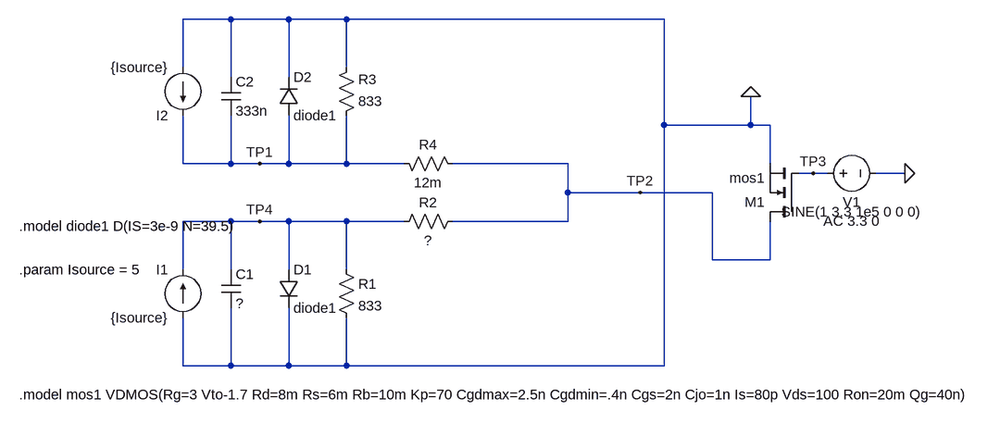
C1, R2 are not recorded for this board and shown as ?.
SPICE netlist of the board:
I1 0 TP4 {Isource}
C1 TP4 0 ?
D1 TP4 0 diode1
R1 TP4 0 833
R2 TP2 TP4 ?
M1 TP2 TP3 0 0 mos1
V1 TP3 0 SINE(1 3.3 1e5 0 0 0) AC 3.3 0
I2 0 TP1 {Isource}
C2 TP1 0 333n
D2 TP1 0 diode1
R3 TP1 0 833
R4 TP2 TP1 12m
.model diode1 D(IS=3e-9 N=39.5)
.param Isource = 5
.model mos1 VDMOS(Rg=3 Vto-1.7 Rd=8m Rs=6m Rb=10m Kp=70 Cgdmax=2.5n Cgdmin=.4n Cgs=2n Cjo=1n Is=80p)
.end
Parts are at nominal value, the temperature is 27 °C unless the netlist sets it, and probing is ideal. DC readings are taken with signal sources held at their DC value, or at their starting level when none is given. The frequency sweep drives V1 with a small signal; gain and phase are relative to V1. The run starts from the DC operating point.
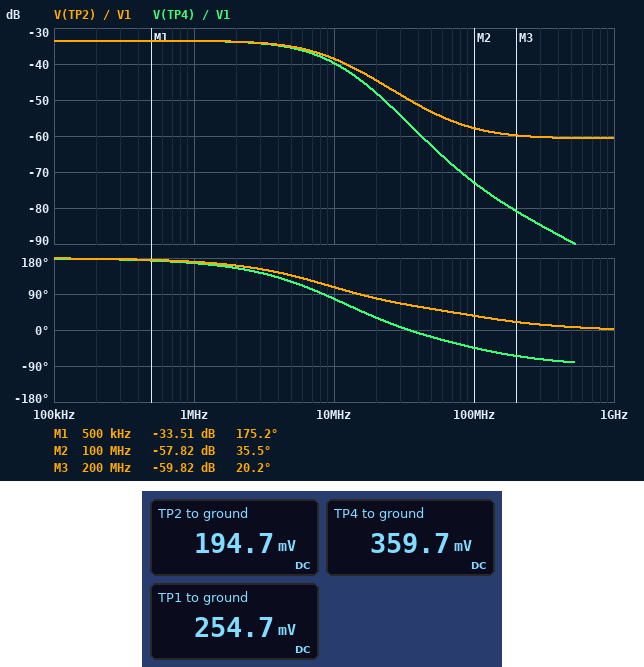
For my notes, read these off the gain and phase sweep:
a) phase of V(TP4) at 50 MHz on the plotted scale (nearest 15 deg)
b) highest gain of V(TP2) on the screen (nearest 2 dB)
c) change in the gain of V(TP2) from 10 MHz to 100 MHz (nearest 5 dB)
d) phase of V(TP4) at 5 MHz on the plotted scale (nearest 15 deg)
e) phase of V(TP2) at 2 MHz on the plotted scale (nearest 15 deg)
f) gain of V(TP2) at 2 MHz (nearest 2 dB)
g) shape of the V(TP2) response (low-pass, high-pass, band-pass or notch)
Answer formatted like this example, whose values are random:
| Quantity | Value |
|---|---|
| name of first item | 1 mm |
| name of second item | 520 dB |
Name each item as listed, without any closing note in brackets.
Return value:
| Quantity | Value |
|---|---|
| phase of V(TP4) at 50 MHz on the plotted scale | -15 deg |
| highest gain of V(TP2) on the screen | -34 dB |
| change in the gain of V(TP2) from 10 MHz to 100 MHz | -20 dB |
| phase of V(TP4) at 5 MHz on the plotted scale | 120 deg |
| phase of V(TP2) at 2 MHz on the plotted scale | 165 deg |
| gain of V(TP2) at 2 MHz | -34 dB |
| shape of the V(TP2) response | low-pass |
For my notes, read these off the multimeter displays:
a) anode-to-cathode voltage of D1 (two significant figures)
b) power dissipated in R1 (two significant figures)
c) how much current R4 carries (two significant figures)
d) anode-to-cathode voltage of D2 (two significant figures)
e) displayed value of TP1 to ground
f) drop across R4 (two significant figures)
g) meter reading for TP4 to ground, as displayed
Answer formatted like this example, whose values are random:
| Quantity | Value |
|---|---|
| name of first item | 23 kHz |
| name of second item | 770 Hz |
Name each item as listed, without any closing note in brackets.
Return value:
| Quantity | Value |
|---|---|
| anode-to-cathode voltage of D1 | 360 mV |
| power dissipated in R1 | 160 µW |
| how much current R4 carries | 5.0 A |
| anode-to-cathode voltage of D2 | 250 mV |
| displayed value of TP1 to ground | 254.7 mV |
| drop across R4 | 60 mV |
| meter reading for TP4 to ground, as displayed | 359.7 mV |
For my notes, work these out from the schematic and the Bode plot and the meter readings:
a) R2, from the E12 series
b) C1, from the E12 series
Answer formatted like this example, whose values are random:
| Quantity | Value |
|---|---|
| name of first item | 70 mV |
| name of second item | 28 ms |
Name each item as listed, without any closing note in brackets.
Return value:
| Quantity | Value |
|---|---|
| R2, from the E12 series | 0.033 Ω |
| C1, from the E12 series | 270 nF |
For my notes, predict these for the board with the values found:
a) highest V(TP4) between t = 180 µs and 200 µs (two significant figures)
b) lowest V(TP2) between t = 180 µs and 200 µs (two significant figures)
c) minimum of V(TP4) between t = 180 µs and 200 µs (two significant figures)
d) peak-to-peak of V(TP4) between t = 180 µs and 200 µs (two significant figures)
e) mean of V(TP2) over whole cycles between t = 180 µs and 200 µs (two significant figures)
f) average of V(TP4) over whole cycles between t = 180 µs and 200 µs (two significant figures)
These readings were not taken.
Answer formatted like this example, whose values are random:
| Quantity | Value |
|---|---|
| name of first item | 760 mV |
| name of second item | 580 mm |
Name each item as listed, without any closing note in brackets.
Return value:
| Quantity | Value |
|---|---|
| highest V(TP4) between t = 180 µs and 200 µs | 22 V |
| lowest V(TP2) between t = 180 µs and 200 µs | 160 mV |
| minimum of V(TP4) between t = 180 µs and 200 µs | 330 mV |
| peak-to-peak of V(TP4) between t = 180 µs and 200 µs | 21 V |
| mean of V(TP2) over whole cycles between t = 180 µs and 200 µs | 5.3 V |
| average of V(TP4) over whole cycles between t = 180 µs and 200 µs | 5.5 V |
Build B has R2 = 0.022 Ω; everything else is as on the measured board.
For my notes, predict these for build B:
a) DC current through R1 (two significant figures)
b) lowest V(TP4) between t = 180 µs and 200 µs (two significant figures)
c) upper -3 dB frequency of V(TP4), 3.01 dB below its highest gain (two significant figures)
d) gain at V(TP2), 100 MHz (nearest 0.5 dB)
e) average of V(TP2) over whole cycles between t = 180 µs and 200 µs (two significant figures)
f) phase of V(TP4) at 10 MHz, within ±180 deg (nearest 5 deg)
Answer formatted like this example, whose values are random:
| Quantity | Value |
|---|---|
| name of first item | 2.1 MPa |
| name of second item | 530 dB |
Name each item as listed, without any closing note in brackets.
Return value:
| Quantity | Value |
|---|---|
| DC current through R1 | 370 µA |
| lowest V(TP4) between t = 180 µs and 200 µs | 270 mV |
| upper -3 dB frequency of V(TP4), 3.01 dB below its highest gain | 6.8 MHz |
| gain at V(TP2), 100 MHz | -58.5 dB |
| average of V(TP2) over whole cycles between t = 180 µs and 200 µs | 5.3 V |
| phase of V(TP4) at 10 MHz, within ±180 deg | 85 deg |
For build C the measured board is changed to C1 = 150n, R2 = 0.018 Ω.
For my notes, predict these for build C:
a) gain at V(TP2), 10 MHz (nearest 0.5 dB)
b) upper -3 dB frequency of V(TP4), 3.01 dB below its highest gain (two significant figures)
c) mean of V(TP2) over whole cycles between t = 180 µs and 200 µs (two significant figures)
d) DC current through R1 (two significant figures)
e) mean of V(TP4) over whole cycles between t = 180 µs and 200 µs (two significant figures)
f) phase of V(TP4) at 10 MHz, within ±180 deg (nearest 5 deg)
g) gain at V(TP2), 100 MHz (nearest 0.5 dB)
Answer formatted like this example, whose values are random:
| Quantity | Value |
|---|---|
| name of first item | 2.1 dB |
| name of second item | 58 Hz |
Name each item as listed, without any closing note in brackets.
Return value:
| Quantity | Value |
|---|---|
| gain at V(TP2), 10 MHz | -37.5 dB |
| upper -3 dB frequency of V(TP4), 3.01 dB below its highest gain | 8.0 MHz |
| mean of V(TP2) over whole cycles between t = 180 µs and 200 µs | 5.5 V |
| DC current through R1 | 340 µA |
| mean of V(TP4) over whole cycles between t = 180 µs and 200 µs | 5.6 V |
| phase of V(TP4) at 10 MHz, within ±180 deg | 100 deg |
| gain at V(TP2), 100 MHz | -58.5 dB |
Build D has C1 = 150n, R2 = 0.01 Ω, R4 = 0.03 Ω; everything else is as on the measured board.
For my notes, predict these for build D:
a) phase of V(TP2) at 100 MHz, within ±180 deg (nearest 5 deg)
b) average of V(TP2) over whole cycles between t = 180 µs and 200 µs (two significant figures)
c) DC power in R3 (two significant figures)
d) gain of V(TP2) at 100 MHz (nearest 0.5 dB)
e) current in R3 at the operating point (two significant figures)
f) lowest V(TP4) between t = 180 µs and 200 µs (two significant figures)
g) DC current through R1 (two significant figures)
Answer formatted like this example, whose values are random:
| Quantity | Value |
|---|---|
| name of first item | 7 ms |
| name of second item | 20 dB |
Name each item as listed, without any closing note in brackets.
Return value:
| Quantity | Value |
|---|---|
| phase of V(TP2) at 100 MHz, within ±180 deg | 25 deg |
| average of V(TP2) over whole cycles between t = 180 µs and 200 µs | 5.5 V |
| DC power in R3 | 140 µW |
| gain of V(TP2) at 100 MHz | -57.0 dB |
| current in R3 at the operating point | 410 µA |
| lowest V(TP4) between t = 180 µs and 200 µs | 210 mV |
| DC current through R1 | 290 µA |
